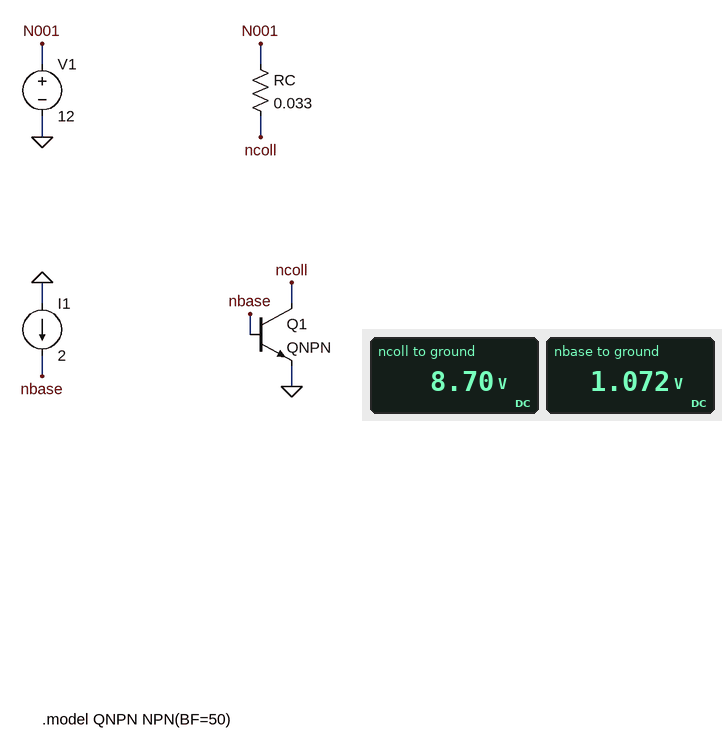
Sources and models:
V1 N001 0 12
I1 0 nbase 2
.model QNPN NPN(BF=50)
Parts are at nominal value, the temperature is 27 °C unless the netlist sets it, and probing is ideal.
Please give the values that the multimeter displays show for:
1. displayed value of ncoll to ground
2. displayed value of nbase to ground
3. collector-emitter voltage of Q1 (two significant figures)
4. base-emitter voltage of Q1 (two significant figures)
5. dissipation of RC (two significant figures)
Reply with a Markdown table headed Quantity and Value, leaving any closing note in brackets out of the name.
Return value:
| Quantity | Value |
|---|---|
| displayed value of ncoll to ground | 8.70 V |
| displayed value of nbase to ground | 1.072 V |
| collector-emitter voltage of Q1 | 8.7 V |
| base-emitter voltage of Q1 | 1.1 V |
| dissipation of RC | 330 W |
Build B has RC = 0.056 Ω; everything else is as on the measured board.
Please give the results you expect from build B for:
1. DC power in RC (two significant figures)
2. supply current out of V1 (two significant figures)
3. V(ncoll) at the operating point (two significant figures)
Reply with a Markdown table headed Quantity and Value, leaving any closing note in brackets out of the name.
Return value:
| Quantity | Value |
|---|---|
| DC power in RC | 560 W |
| supply current out of V1 | 100 A |
| V(ncoll) at the operating point | 6.4 V |
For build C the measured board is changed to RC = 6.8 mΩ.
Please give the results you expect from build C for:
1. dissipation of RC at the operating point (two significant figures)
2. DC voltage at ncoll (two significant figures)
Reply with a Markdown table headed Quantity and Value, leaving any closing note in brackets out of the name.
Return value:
| Quantity | Value |
|---|---|
| dissipation of RC at the operating point | 68 W |
| DC voltage at ncoll | 11 V |
